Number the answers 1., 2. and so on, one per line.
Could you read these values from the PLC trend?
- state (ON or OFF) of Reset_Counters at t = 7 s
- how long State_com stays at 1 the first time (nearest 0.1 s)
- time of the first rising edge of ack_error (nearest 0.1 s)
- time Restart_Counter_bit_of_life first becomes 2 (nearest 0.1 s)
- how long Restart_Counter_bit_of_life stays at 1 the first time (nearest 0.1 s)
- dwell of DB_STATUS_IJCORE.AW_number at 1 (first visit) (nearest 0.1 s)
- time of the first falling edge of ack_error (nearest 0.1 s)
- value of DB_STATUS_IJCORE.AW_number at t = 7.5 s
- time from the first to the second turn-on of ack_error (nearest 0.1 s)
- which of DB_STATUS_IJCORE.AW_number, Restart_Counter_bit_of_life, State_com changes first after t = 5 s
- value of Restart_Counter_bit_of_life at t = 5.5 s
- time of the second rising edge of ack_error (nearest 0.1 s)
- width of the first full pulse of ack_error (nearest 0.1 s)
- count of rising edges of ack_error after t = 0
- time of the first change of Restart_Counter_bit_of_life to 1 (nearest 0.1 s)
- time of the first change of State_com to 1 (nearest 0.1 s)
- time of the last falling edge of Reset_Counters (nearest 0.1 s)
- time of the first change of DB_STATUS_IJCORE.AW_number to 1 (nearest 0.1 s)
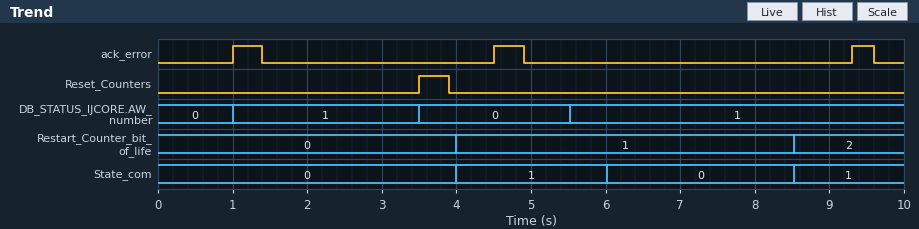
1. OFF
2. 2.0 s
3. 1.0 s
4. 8.5 s
5. 4.5 s
6. 2.5 s
7. 1.4 s
8. 1
9. 3.5 s
10. DB_STATUS_IJCORE.AW_number
11. 1
12. 4.5 s
13. 0.4 s
14. 3
15. 4.0 s
16. 4.0 s
17. 3.9 s
18. 1.0 s
